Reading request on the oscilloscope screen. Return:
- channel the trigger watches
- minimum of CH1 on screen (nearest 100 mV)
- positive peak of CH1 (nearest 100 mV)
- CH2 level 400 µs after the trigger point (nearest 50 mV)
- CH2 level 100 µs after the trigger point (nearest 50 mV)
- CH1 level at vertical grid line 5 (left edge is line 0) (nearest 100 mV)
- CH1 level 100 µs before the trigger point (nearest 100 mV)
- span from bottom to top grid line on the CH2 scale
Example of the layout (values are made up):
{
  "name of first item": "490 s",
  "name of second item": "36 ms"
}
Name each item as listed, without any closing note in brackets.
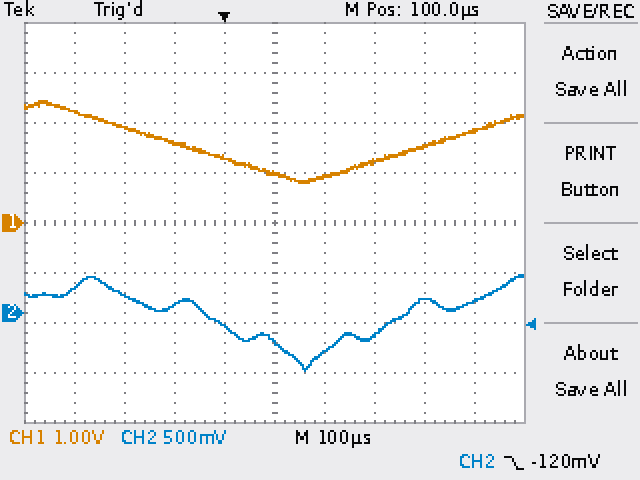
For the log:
{
  "channel the trigger watches": "CH2",
  "minimum of CH1 on screen": "800 mV",
  "positive peak of CH1": "2.4 V",
  "CH2 level 400 µs after the trigger point": "150 mV",
  "CH2 level 100 µs after the trigger point": "-300 mV",
  "CH1 level at vertical grid line 5 (left edge is line 0)": "1.0 V",
  "CH1 level 100 µs before the trigger point": "1.6 V",
  "span from bottom to top grid line on the CH2 scale": "4 V"
}
